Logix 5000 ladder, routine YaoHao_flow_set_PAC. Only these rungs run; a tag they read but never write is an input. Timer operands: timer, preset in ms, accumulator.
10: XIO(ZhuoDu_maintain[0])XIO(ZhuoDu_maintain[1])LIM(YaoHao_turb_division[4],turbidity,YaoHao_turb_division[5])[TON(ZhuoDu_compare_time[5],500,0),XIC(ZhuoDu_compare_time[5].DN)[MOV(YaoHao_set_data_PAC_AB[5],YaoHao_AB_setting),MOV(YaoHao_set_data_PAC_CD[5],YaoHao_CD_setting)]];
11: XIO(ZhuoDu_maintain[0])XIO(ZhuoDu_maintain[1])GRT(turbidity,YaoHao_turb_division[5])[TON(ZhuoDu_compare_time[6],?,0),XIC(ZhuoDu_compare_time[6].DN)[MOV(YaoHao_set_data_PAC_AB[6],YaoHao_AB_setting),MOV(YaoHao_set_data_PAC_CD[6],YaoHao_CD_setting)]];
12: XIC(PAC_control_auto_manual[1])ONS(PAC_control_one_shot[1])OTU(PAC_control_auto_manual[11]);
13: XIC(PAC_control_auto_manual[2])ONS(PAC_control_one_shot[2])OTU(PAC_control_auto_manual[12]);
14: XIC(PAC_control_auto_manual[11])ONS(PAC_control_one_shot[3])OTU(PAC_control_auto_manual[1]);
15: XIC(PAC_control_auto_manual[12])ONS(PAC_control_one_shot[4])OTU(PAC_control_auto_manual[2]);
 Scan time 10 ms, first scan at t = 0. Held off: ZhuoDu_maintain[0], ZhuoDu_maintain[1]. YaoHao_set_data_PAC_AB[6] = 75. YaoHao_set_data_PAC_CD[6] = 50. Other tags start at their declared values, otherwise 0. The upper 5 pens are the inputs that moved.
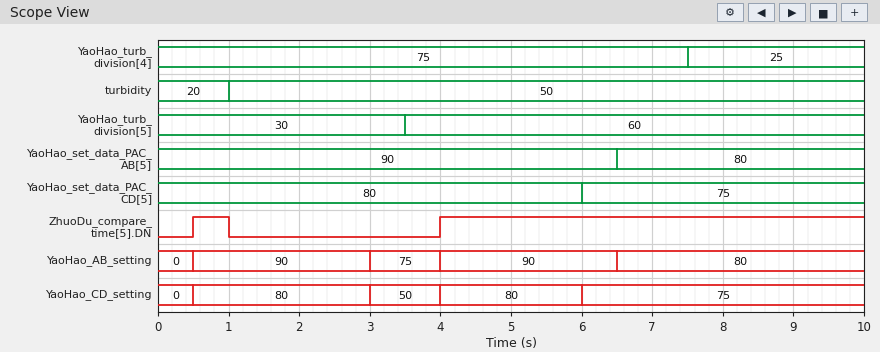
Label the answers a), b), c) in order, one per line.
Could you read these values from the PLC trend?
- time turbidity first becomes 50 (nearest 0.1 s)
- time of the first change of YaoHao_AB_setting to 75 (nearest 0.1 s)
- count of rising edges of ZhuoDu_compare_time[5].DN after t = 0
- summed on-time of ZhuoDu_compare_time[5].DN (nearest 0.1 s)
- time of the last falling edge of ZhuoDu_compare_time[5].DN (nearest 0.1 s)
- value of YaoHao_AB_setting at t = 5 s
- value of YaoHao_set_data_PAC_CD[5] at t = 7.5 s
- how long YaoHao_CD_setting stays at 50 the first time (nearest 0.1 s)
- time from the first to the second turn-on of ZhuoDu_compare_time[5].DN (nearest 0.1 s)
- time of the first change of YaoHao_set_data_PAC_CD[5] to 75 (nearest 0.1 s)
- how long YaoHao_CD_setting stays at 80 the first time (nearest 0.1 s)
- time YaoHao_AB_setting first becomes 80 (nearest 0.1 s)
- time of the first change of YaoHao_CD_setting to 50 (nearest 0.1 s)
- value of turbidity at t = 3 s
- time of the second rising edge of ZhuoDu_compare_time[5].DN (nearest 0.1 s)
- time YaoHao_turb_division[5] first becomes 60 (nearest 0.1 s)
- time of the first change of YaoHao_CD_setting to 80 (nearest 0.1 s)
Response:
a) 1.0 s
b) 3.0 s
c) 2
d) 6.5 s
e) 1.0 s
f) 90
g) 75
h) 1.0 s
i) 3.5 s
j) 6.0 s
k) 2.5 s
l) 6.5 s
m) 3.0 s
n) 50
o) 4.0 s
p) 3.5 s
q) 0.5 s
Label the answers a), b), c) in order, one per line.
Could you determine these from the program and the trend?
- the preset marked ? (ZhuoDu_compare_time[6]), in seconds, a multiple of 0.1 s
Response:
a) 2.0 s
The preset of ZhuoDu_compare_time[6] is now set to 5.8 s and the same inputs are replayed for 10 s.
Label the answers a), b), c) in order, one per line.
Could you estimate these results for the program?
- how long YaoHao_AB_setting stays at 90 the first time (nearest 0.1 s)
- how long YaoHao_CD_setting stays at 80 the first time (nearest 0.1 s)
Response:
a) 6.0 s
b) 5.5 s
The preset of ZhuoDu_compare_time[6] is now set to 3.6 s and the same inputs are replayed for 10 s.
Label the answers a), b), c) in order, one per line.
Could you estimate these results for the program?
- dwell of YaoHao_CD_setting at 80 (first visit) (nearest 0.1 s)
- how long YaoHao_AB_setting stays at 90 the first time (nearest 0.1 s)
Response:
a) 5.5 s
b) 6.0 s
